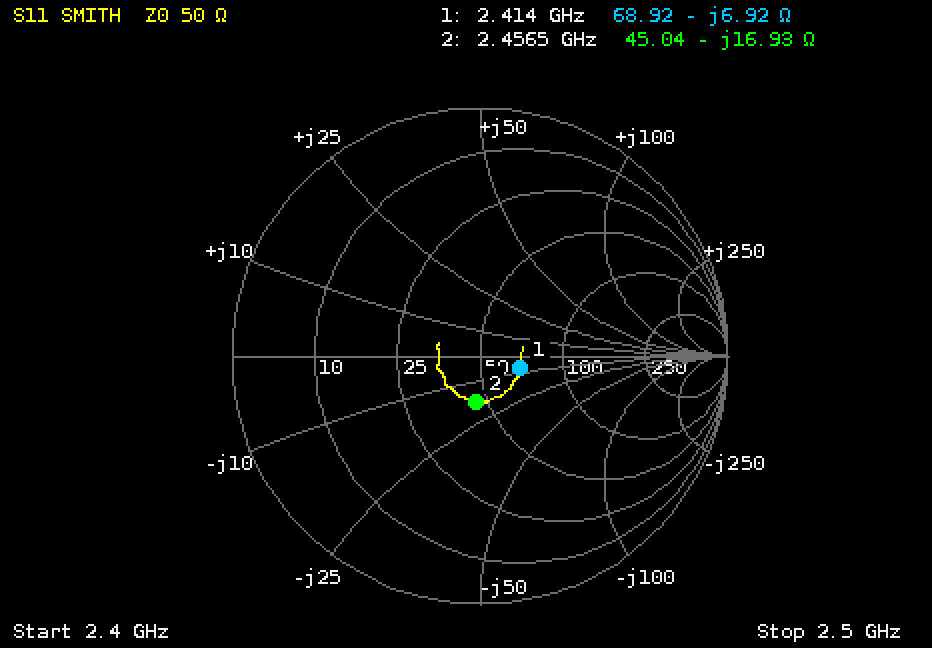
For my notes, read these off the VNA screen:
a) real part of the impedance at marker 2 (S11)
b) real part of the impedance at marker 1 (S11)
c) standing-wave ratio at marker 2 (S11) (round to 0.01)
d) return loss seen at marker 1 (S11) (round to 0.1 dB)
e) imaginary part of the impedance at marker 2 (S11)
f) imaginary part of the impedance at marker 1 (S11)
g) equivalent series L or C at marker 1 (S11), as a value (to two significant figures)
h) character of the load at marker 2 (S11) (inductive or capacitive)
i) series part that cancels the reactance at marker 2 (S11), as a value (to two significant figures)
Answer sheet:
45.04 Ω
68.92 Ω
1.45
15.4 dB
-16.93 Ω
-6.92 Ω
9.5 pF
capacitive
1.1 nH
